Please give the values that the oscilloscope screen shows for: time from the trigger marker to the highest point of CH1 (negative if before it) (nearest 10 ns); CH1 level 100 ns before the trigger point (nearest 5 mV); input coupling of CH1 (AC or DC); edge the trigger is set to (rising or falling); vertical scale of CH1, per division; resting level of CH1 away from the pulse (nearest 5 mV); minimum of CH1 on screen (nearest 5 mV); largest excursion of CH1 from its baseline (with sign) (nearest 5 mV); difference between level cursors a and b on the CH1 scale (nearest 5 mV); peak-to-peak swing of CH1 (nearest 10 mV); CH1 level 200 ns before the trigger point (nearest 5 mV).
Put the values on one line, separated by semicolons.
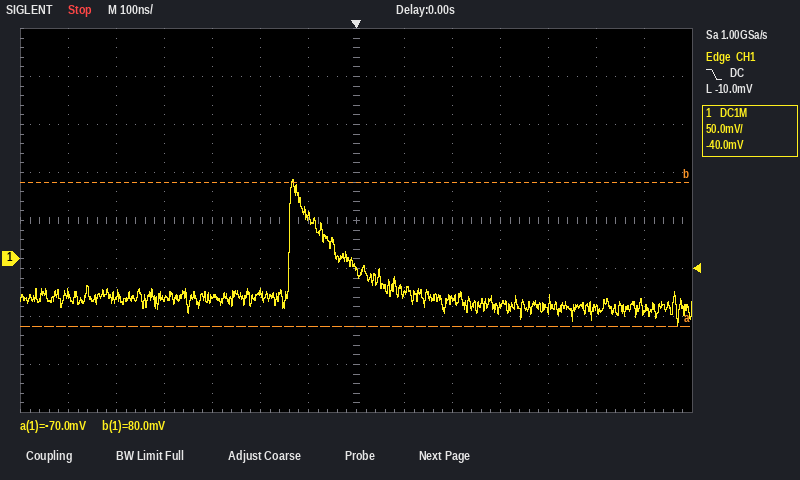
-130 ns; 45 mV; DC; falling; 50 mV; -40 mV; -70 mV; +125 mV; 150 mV; 150 mV; -35 mV
